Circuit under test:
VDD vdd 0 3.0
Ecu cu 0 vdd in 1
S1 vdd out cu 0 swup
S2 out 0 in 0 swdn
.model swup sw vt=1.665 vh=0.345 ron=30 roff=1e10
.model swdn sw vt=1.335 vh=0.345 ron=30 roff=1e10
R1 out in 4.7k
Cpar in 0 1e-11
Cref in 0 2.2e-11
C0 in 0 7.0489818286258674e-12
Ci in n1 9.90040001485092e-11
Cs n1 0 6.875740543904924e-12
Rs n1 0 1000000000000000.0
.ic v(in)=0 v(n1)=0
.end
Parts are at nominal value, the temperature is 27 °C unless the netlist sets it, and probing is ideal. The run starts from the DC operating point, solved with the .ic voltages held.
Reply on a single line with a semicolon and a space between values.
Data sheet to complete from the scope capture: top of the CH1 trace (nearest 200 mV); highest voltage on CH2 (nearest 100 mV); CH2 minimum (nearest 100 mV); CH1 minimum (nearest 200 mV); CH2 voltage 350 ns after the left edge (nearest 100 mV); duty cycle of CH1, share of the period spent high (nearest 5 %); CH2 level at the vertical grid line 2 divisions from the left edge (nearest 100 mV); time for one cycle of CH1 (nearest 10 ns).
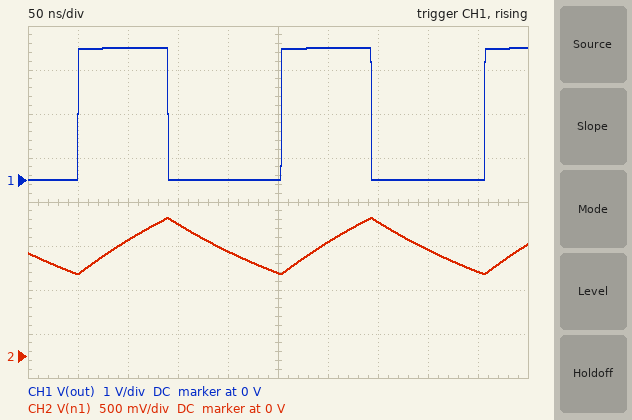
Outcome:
3.0 V; 1.6 V; 900 mV; 0 V; 1.5 V; 45 %; 1.3 V; 200 ns
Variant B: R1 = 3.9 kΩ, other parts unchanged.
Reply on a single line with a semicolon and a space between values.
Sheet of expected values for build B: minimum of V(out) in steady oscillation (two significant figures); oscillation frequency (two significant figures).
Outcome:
7.6 mV; 5.9 MHz
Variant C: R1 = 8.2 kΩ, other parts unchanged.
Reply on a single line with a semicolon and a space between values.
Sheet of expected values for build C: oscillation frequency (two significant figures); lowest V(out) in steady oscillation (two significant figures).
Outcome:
2.8 MHz; 3.6 mV
